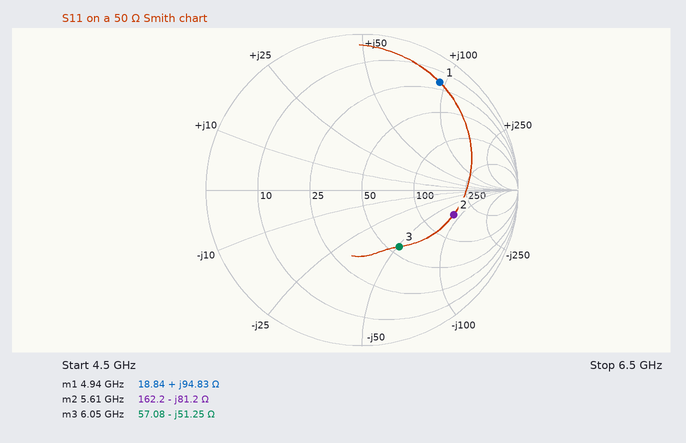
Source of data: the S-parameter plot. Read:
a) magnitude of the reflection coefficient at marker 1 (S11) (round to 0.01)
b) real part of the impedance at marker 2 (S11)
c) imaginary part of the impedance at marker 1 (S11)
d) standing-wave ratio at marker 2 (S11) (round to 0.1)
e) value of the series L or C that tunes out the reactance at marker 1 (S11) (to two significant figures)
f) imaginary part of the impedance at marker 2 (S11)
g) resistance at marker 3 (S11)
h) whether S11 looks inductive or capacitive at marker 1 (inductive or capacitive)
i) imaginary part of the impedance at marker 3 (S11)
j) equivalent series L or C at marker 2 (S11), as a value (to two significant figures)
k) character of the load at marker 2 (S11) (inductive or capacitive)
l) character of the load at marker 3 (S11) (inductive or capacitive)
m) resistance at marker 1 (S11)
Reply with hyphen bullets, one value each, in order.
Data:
- 0.85
- 162.2 Ω
- +94.83 Ω
- 4.1
- 340 fF
- -81.2 Ω
- 57.08 Ω
- inductive
- -51.25 Ω
- 350 fF
- capacitive
- capacitive
- 18.84 Ω
